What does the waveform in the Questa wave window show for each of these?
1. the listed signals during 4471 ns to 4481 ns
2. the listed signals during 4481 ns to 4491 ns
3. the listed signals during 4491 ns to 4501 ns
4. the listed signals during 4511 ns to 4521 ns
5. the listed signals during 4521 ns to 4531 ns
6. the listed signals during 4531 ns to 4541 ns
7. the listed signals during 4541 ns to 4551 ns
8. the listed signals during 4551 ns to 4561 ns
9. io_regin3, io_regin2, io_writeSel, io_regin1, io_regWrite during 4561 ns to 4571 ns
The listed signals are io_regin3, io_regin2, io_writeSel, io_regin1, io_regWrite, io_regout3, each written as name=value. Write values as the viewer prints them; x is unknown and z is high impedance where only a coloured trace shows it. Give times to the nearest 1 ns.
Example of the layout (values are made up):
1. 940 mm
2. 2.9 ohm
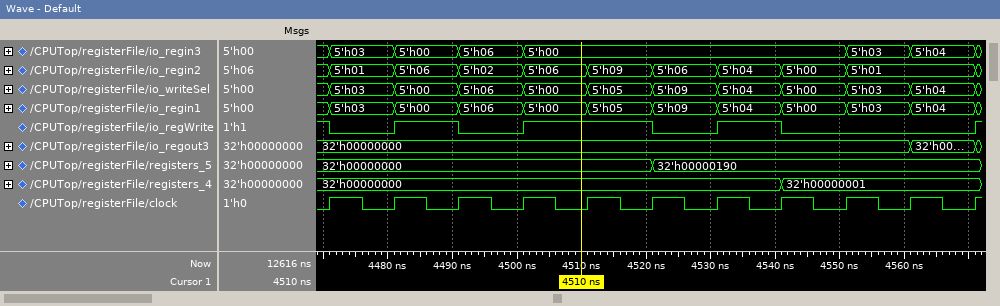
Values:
1. io_regin3=5'h03, io_regin2=5'h01, io_writeSel=5'h03, io_regin1=5'h03, io_regWrite=0, io_regout3=32'h00000000
2. io_regin3=5'h00, io_regin2=5'h06, io_writeSel=5'h00, io_regin1=5'h00, io_regWrite=1, io_regout3=32'h00000000
3. io_regin3=5'h06, io_regin2=5'h02, io_writeSel=5'h06, io_regin1=5'h06, io_regWrite=0, io_regout3=32'h00000000
4. io_regin3=5'h00, io_regin2=5'h09, io_writeSel=5'h05, io_regin1=5'h05, io_regWrite=1, io_regout3=32'h00000000
5. io_regin3=5'h00, io_regin2=5'h06, io_writeSel=5'h09, io_regin1=5'h09, io_regWrite=0, io_regout3=32'h00000000
6. io_regin3=5'h00, io_regin2=5'h04, io_writeSel=5'h04, io_regin1=5'h04, io_regWrite=1, io_regout3=32'h00000000
7. io_regin3=5'h00, io_regin2=5'h00, io_writeSel=5'h00, io_regin1=5'h00, io_regWrite=0, io_regout3=32'h00000000
8. io_regin3=5'h03, io_regin2=5'h01, io_writeSel=5'h03, io_regin1=5'h03, io_regWrite=0, io_regout3=32'h00000000
9. io_regin3=5'h04, io_regin2=5'h01, io_writeSel=5'h04, io_regin1=5'h04, io_regWrite=0
